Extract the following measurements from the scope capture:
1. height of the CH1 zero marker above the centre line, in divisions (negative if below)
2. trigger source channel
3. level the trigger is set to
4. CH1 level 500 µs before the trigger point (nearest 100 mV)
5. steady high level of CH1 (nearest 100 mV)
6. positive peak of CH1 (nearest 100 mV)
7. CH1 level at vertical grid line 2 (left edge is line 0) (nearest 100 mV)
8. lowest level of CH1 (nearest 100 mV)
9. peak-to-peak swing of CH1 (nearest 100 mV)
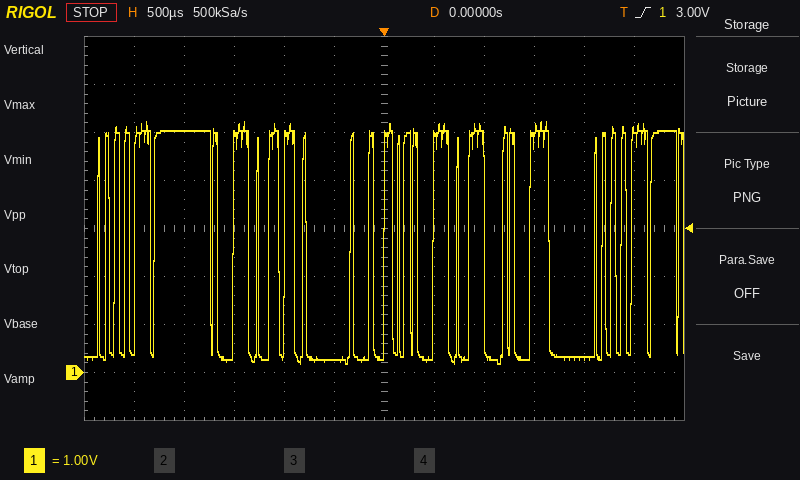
-3.0 div
CH1
3.00 V
300 mV
5.0 V
5.2 V
5.0 V
200 mV
5.0 V
